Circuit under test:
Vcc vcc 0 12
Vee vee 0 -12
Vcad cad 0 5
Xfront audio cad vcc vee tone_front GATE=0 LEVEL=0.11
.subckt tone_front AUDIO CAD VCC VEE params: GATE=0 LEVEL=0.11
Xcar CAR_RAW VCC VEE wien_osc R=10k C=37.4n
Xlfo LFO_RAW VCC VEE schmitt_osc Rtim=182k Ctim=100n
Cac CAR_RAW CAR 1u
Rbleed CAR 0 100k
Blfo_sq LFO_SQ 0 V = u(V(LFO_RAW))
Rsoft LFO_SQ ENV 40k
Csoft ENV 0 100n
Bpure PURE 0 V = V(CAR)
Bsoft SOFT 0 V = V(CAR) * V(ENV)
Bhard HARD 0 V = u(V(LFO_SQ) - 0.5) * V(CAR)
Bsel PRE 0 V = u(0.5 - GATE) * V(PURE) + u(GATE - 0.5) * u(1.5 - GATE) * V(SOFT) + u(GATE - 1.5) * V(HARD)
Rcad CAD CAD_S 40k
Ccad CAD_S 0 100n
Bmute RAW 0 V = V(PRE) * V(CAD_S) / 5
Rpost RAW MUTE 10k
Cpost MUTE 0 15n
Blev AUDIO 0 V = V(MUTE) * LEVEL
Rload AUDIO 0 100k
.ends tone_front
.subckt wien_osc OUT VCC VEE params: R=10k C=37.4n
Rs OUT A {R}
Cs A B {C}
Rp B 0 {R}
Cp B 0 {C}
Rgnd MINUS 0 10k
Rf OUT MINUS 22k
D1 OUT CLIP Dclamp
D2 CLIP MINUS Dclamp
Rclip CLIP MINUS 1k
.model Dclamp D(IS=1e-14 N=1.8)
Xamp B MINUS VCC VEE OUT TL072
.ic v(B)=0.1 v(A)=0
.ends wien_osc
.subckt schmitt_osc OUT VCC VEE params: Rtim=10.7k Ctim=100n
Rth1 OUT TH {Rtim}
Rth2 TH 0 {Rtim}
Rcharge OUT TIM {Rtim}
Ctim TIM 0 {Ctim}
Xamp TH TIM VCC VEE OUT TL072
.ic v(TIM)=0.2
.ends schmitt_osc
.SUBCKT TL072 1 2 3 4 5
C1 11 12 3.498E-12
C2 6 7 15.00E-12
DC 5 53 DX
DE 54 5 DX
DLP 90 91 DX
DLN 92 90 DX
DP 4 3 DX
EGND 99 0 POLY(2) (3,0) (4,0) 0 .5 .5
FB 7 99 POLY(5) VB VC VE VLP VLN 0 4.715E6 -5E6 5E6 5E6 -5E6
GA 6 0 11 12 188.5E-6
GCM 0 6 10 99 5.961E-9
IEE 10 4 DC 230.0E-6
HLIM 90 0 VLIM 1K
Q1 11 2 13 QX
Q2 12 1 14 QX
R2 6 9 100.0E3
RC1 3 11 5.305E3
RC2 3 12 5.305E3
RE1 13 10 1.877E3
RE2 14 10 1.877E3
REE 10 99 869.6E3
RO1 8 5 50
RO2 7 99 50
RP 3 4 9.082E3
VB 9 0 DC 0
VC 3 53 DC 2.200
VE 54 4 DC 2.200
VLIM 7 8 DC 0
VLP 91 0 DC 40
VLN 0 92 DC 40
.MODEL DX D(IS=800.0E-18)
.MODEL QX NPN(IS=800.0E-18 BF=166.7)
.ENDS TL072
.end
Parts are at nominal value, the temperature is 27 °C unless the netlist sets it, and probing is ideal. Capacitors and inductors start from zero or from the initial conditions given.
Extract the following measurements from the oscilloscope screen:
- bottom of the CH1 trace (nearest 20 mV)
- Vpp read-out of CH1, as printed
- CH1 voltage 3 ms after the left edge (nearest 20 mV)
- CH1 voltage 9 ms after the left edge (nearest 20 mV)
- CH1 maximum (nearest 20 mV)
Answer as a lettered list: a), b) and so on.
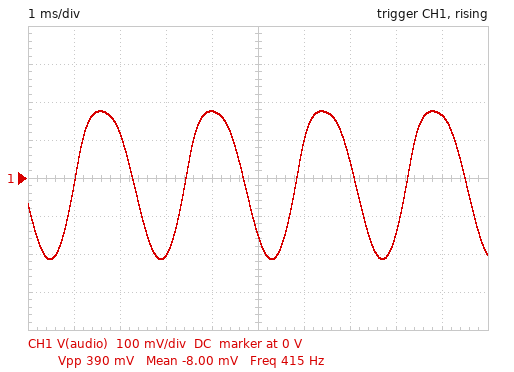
a) -220 mV
b) 390 mV
c) -200 mV
d) 160 mV
e) 180 mV
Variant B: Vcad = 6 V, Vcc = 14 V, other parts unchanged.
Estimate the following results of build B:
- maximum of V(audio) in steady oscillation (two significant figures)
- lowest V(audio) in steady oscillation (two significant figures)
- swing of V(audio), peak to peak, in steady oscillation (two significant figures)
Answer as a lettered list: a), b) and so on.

a) 210 mV
b) -260 mV
c) 470 mV
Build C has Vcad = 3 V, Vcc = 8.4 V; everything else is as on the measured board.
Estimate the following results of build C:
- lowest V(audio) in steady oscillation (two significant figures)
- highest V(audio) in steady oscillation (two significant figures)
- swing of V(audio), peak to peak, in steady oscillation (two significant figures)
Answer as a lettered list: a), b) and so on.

a) -130 mV
b) 110 mV
c) 230 mV
